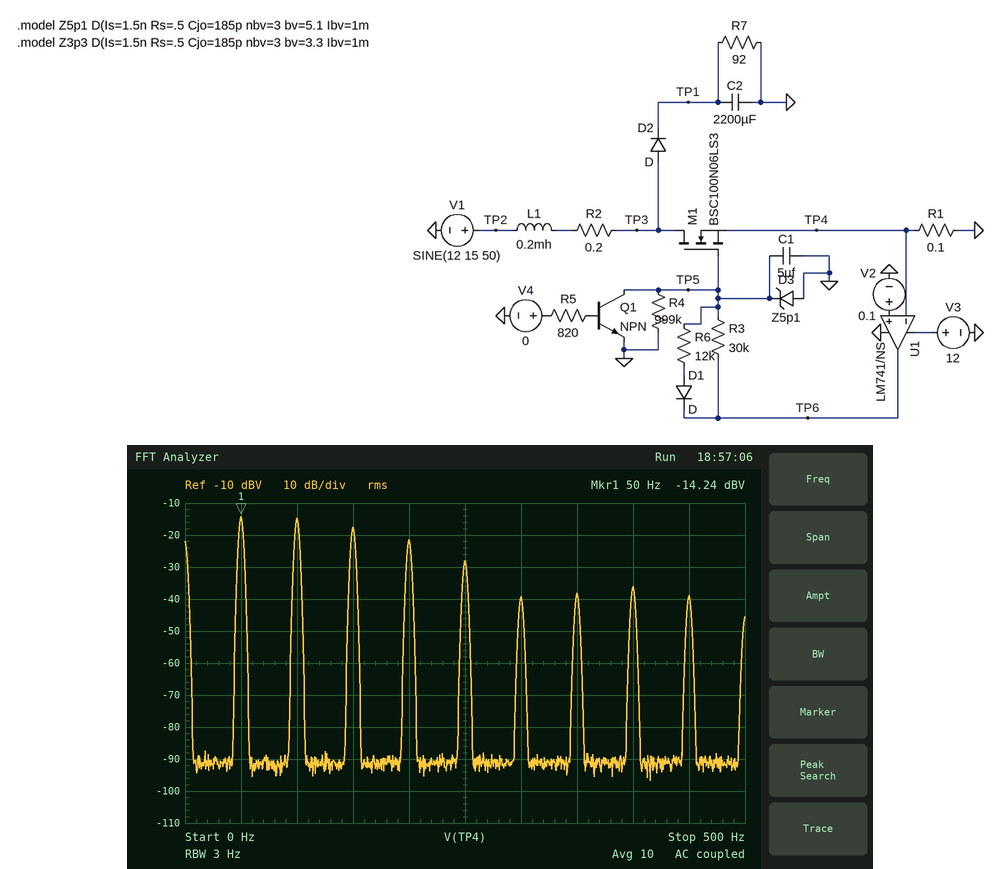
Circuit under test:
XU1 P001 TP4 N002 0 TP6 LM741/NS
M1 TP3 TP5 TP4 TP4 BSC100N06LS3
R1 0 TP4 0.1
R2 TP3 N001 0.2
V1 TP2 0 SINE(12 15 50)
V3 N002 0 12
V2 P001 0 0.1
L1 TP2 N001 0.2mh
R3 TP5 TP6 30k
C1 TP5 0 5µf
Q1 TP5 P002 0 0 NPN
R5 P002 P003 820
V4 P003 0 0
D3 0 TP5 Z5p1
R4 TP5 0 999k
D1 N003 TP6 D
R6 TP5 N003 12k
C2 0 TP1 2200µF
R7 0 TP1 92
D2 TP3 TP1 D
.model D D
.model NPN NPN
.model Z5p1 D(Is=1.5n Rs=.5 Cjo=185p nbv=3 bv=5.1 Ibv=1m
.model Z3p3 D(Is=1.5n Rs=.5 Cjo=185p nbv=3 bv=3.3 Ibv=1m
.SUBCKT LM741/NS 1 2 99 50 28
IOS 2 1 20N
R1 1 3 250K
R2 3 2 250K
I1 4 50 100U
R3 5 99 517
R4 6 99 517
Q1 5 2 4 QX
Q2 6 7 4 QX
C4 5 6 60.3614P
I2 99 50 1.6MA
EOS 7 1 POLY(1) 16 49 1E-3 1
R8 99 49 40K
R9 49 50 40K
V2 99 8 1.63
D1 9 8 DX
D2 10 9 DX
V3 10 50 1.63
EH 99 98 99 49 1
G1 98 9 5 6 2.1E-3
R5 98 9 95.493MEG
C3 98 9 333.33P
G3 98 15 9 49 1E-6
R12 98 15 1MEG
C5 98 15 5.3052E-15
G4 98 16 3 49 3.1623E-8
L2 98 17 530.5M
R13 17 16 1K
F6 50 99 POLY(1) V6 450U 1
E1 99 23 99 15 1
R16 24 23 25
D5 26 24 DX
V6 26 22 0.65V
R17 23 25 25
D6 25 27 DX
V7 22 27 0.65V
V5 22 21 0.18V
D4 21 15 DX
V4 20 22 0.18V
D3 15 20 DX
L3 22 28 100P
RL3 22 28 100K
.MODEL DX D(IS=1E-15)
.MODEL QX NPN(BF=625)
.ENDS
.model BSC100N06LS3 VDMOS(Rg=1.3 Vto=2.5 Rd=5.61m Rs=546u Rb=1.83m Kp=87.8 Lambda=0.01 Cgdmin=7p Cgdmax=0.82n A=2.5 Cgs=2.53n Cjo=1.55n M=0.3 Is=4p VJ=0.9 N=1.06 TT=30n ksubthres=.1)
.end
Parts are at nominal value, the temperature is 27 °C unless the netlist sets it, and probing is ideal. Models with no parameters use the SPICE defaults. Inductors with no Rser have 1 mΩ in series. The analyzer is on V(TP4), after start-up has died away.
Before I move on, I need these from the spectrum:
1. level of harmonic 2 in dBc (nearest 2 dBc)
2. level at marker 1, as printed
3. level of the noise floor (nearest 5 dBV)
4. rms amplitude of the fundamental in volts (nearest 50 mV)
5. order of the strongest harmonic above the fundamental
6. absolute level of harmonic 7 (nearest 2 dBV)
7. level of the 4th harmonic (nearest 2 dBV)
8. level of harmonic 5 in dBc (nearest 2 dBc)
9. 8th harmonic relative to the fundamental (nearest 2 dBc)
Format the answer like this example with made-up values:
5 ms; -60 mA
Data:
0 dBc; -14.24 dBV; -90 dBV; 200 mV; 2; -38 dBV; -22 dBV; -14 dBc; -22 dBc
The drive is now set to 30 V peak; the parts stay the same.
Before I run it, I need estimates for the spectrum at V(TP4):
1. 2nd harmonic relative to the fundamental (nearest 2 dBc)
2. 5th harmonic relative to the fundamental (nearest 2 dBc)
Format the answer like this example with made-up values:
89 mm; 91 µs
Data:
-4 dBc; -22 dBc
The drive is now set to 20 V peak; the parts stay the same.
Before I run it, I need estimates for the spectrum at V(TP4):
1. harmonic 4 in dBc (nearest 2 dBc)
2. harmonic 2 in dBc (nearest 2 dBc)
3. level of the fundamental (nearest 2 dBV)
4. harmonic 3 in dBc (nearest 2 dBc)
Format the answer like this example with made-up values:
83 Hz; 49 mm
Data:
-18 dBc; -2 dBc; -4 dBV; -8 dBc
